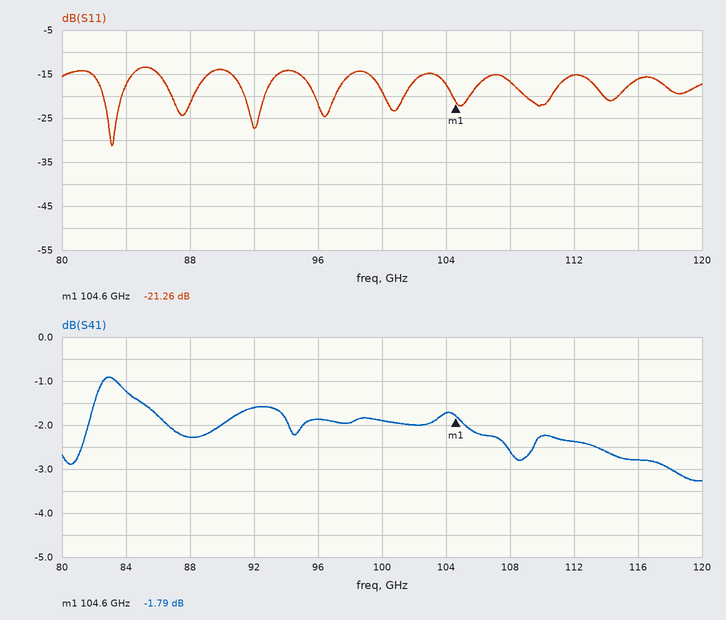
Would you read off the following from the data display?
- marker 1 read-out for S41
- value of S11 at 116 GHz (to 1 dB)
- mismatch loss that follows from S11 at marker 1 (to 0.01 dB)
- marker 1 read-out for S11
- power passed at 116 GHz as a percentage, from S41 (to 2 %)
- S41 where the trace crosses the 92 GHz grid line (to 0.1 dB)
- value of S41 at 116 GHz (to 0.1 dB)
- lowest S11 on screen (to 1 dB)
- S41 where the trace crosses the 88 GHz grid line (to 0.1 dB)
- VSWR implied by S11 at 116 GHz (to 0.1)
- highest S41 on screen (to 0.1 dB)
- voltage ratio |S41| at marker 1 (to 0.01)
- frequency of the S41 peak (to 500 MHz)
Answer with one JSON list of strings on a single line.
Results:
["-1.79 dB", "-16 dB", "0.03 dB", "-21.26 dB", "52 %", "-1.6 dB", "-2.8 dB", "-31 dB", "-2.3 dB", "1.4", "-0.9 dB", "0.81", "83.0 GHz"]
